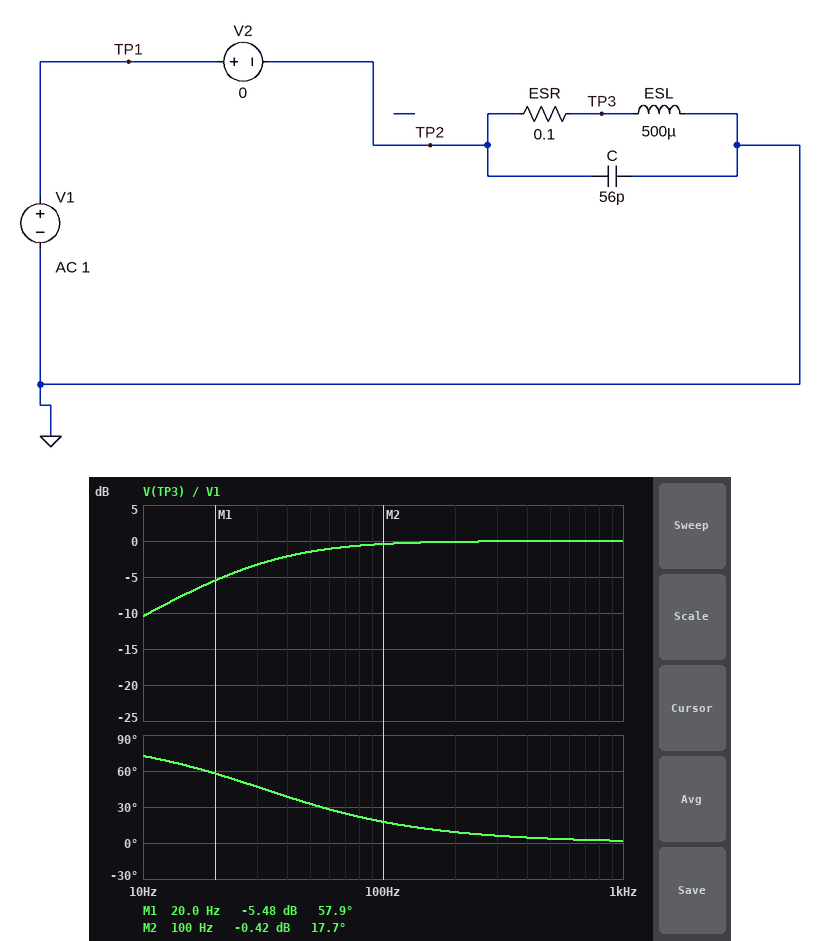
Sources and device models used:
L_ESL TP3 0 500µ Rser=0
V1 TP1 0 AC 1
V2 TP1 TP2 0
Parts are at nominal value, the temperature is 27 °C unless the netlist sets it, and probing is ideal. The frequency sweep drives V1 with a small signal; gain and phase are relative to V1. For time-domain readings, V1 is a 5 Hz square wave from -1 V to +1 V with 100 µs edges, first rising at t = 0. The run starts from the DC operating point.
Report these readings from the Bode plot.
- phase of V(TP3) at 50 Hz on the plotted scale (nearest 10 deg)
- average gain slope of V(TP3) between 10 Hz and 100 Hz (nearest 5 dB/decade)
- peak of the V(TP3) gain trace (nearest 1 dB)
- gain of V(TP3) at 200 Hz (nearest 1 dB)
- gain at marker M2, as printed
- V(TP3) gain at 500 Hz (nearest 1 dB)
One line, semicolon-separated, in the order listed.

30 deg; 10 dB/decade; 0 dB; 0 dB; -0.42 dB; 0 dB
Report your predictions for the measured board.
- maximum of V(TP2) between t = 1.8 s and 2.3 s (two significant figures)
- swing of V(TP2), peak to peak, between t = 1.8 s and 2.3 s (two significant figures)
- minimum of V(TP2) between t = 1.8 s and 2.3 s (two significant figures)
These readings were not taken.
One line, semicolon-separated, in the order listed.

1.0 V; 2.0 V; -1.0 V
